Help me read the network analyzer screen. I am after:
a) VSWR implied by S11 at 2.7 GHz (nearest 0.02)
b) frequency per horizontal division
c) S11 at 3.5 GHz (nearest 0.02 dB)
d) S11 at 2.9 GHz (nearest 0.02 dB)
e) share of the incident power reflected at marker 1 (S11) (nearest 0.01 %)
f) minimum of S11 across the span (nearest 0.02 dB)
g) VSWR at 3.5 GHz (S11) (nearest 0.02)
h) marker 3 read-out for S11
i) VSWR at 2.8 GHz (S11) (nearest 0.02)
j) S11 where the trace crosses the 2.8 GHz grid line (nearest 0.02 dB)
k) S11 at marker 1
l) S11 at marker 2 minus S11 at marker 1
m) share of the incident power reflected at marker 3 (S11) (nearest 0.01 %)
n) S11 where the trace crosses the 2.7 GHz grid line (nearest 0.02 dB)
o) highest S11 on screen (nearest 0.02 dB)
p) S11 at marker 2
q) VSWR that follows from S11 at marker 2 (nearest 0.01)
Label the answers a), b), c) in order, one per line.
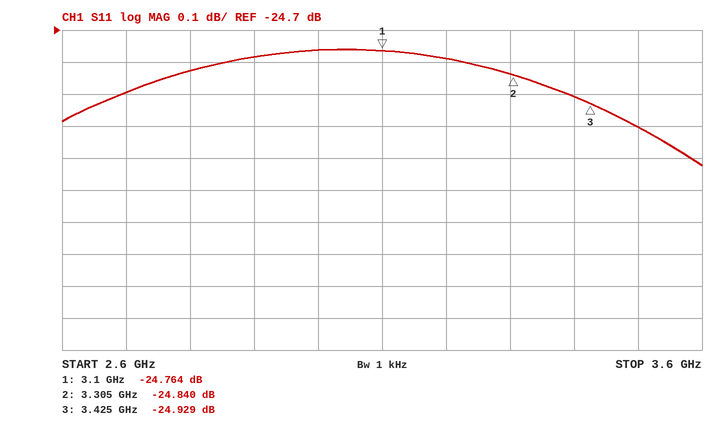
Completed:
a) 1.12
b) 100 MHz
c) -25.00 dB
d) -24.78 dB
e) 0.33 %
f) -25.12 dB
g) 1.12
h) -24.929 dB
i) 1.12
j) -24.82 dB
k) -24.764 dB
l) -0.076 dB
m) 0.32 %
n) -24.90 dB
o) -24.76 dB
p) -24.840 dB
q) 1.12
